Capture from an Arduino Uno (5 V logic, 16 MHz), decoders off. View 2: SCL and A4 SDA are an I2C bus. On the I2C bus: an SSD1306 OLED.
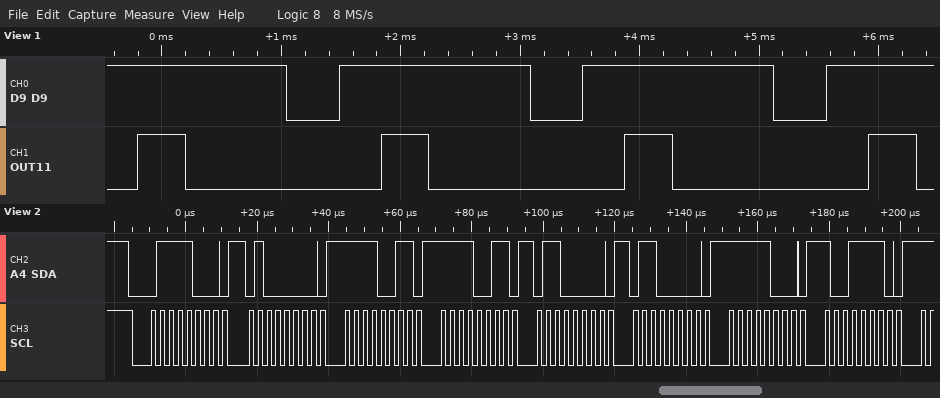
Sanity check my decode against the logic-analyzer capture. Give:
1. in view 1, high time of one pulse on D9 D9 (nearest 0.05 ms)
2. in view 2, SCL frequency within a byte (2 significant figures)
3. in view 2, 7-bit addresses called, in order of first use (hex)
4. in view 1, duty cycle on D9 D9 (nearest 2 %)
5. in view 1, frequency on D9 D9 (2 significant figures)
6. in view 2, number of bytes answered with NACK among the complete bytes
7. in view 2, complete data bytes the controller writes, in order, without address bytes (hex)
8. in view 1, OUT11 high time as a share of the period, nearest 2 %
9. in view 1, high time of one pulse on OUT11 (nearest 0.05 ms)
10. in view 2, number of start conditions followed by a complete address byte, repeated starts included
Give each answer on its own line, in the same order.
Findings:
1.60 ms
400 kHz
0x3C
78 %
490 Hz
0
40 F3 F3 60 60 F8 9E
20 %
0.40 ms
1
